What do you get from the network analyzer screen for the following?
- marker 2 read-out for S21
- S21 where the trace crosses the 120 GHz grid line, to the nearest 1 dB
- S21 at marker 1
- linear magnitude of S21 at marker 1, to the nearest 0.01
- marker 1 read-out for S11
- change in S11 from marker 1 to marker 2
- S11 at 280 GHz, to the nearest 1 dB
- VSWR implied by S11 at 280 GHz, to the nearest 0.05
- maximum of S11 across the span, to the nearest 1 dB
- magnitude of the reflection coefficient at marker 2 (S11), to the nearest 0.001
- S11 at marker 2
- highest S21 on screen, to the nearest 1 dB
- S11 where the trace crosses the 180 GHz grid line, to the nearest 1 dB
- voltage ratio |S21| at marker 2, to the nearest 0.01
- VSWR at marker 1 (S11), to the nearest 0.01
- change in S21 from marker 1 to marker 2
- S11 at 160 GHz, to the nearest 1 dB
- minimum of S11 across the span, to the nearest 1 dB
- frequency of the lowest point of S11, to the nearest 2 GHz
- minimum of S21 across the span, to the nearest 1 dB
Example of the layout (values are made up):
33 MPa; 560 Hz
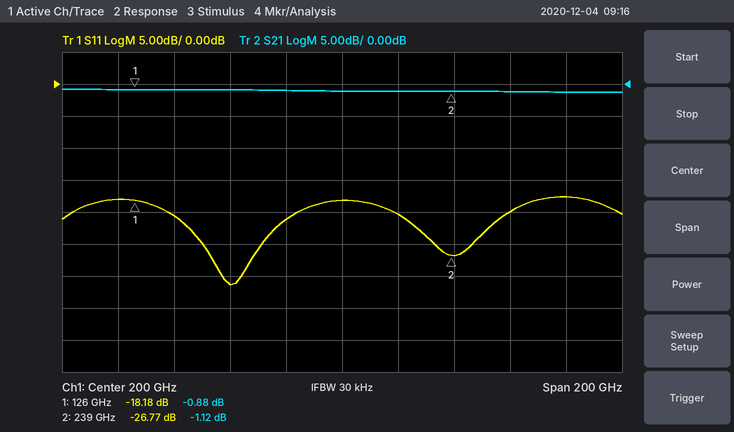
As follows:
-1.12 dB; -1 dB; -0.88 dB; 0.90; -18.18 dB; -8.59 dB; -18 dB; 1.30; -18 dB; 0.046; -26.77 dB; -1 dB; -21 dB; 0.88; 1.28; -0.24 dB; -31 dB; -31 dB; 160 GHz; -1 dB
